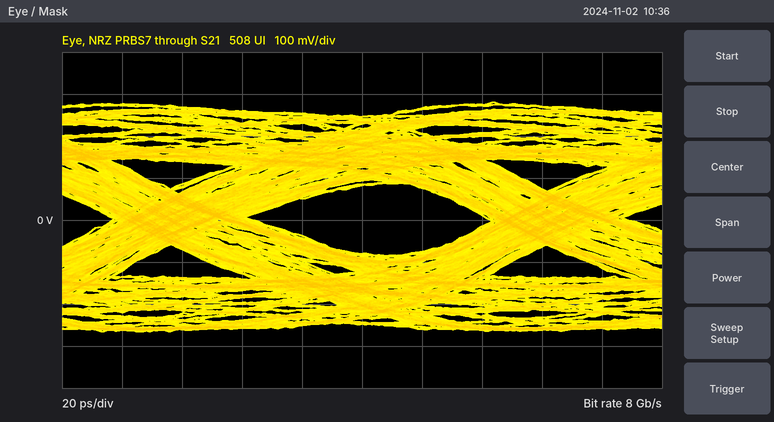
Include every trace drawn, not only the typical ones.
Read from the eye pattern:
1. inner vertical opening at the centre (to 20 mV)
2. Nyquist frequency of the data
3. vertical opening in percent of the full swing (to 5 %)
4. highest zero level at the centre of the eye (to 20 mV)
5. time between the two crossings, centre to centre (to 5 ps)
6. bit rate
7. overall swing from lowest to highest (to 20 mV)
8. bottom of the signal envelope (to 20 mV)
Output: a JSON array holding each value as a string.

["160 mV", "4 GHz", "30 %", "-80 mV", "125 ps", "8 Gb/s", "540 mV", "-260 mV"]
